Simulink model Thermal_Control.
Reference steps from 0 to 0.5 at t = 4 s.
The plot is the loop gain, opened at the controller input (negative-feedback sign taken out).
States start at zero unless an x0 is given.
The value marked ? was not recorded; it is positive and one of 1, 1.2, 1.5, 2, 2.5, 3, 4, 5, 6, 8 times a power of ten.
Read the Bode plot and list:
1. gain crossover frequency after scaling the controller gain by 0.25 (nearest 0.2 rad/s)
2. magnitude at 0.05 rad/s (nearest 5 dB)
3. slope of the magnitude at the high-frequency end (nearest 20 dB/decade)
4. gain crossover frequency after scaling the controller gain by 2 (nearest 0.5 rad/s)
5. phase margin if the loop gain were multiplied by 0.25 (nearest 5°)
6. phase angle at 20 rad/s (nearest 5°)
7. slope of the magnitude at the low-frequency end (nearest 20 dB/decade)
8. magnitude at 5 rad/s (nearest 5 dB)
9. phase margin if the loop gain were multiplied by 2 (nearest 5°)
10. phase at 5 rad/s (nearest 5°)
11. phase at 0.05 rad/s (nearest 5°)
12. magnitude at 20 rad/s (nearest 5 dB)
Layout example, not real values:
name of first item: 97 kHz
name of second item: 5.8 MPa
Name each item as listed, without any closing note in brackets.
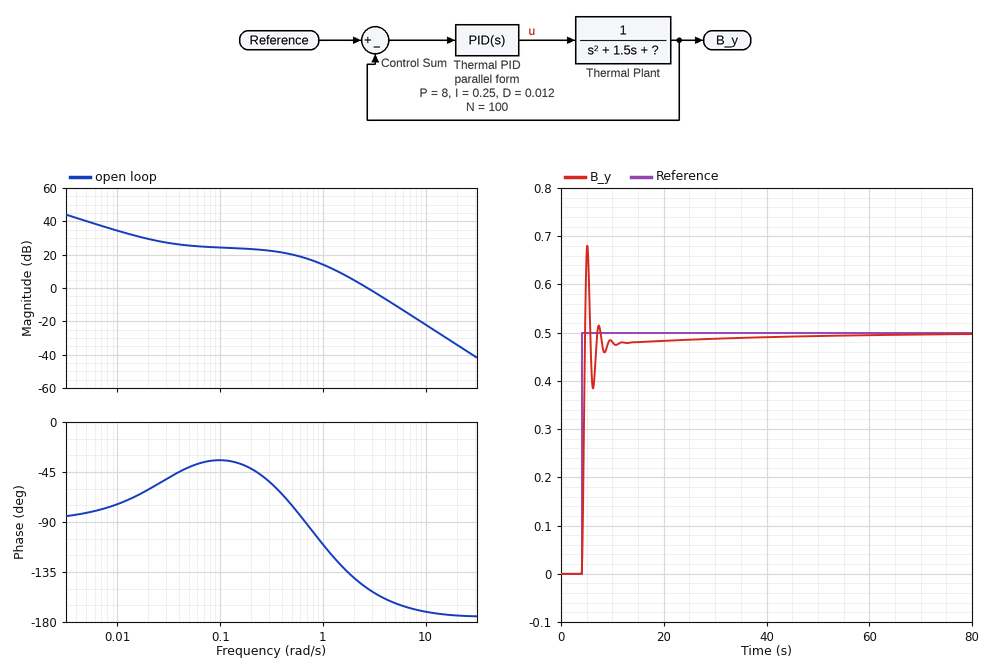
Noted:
gain crossover frequency after scaling the controller gain by 0.25: 1.2 rad/s
magnitude at 0.05 rad/s: 25 dB
slope of the magnitude at the high-frequency end: -40 dB/decade
gain crossover frequency after scaling the controller gain by 2: 4.0 rad/s
phase margin if the loop gain were multiplied by 0.25: 60°
phase angle at 20 rad/s: -175°
slope of the magnitude at the low-frequency end: -20 dB/decade
magnitude at 5 rad/s: -10 dB
phase margin if the loop gain were multiplied by 2: 20°
phase at 5 rad/s: -165°
phase at 0.05 rad/s: -40°
magnitude at 20 rad/s: -35 dB
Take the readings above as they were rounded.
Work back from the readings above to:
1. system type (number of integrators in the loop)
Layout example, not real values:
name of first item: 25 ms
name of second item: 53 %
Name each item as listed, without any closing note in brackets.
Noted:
system type: 1
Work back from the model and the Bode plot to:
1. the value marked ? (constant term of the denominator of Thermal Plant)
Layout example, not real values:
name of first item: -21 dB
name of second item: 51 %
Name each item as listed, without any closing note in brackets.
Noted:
the value marked ?: 0.5
